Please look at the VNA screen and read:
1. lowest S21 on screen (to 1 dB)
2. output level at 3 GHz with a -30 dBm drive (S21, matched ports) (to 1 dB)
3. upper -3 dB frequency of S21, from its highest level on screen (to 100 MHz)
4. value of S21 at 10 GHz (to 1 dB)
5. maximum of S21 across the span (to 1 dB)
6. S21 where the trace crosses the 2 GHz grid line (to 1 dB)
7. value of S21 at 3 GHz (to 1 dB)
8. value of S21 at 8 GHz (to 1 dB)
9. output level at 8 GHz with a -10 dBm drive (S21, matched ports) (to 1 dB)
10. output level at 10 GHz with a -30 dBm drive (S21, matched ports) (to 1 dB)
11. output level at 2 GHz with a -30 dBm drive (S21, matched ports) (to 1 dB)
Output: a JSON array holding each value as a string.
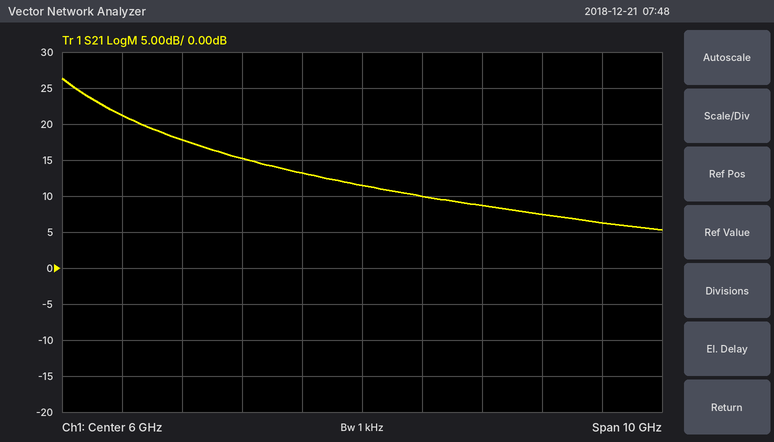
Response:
["5 dB", "-12 dBm", "1.5 GHz", "6 dB", "26 dB", "21 dB", "18 dB", "9 dB", "-1 dBm", "-24 dBm", "-9 dBm"]
